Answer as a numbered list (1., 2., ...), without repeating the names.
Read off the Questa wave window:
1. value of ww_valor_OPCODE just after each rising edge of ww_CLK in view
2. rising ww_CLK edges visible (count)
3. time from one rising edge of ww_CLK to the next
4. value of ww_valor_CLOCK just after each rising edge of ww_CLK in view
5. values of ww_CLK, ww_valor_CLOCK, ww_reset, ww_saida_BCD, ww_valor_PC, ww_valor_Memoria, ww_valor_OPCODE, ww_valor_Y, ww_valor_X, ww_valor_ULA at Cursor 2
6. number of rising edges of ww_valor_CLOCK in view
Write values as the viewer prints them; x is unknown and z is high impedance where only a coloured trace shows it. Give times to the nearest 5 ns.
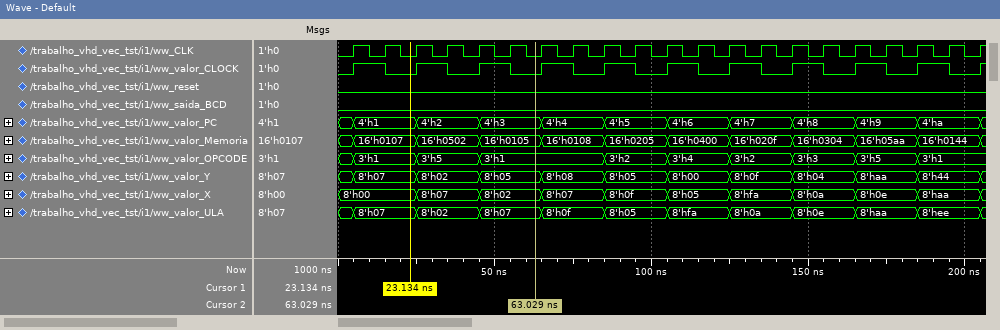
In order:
1. 3'h1, 3'h1, 3'h5, 3'h5, 3'h1, 3'h1, 3'h1, 3'h1, 3'h2, 3'h2, 3'h4, 3'h4, 3'h2, 3'h2, 3'h3, 3'h3, 3'h5, 3'h5, 3'h1, 3'h1, 3'h1
2. 21
3. 10 ns
4. 1 0 1 0 1 0 1 0 1 0 1 0 1 0 1 0 1 0 1 0 1
5. ww_CLK=0, ww_valor_CLOCK=0, ww_reset=0, ww_saida_BCD=0, ww_valor_PC=4'h3, ww_valor_Memoria=16'h0105, ww_valor_OPCODE=3'h1, ww_valor_Y=8'h05, ww_valor_X=8'h02, ww_valor_ULA=8'h07
6. 11
